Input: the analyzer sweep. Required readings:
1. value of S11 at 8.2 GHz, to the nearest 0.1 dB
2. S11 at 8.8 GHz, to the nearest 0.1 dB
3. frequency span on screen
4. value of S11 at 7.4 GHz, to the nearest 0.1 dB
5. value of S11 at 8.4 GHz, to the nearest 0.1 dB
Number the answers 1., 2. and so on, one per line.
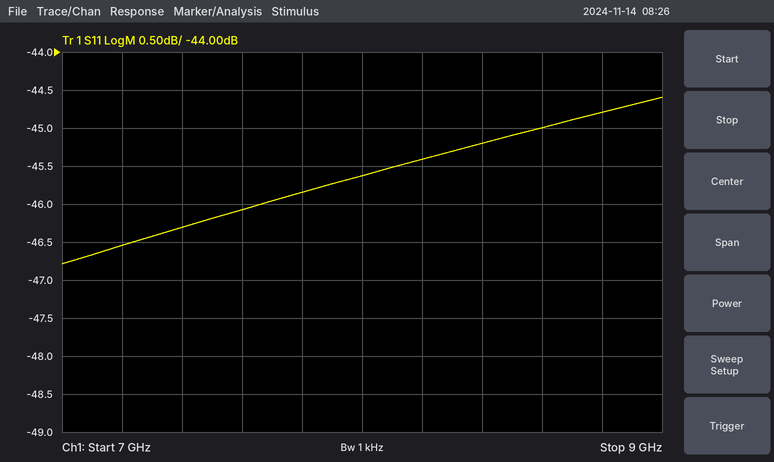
1. -45.4 dB
2. -44.8 dB
3. 2 GHz
4. -46.3 dB
5. -45.2 dB
